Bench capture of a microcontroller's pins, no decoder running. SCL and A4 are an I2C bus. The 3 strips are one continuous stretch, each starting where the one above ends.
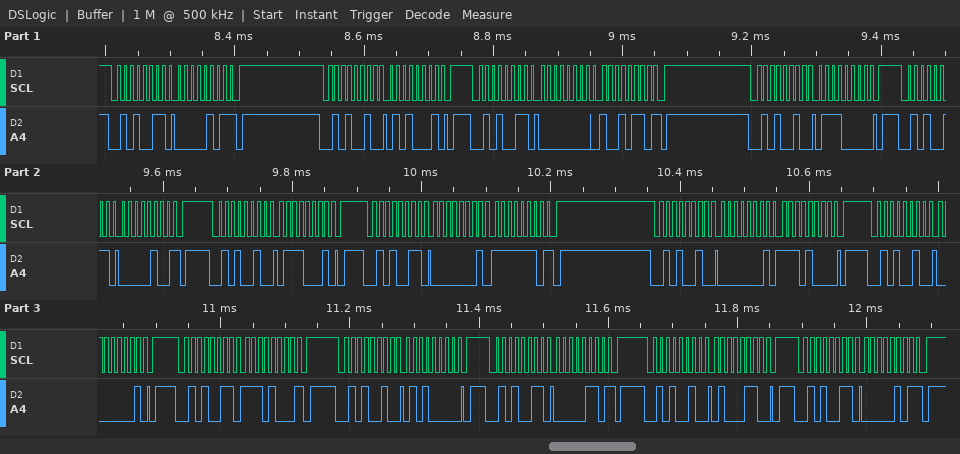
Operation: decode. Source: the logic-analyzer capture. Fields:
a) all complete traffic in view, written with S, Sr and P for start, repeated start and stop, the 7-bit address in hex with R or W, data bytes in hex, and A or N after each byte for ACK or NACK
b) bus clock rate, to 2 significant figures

S 29R A 05 N P S 29W A 51 A P S 29R A 00 A 96 N P S 29W A 70 A P S 29R A 04 N P S 29W A 71 A P S 29R A 01 A FE N P S 29W A 01 A E8 A P S 29W A 01 A P S 29R A E8 N P S 29W A 50 A P S 29R A 06 N P S 29W A 46 A P S 29R A 05 N P
100 kHz
